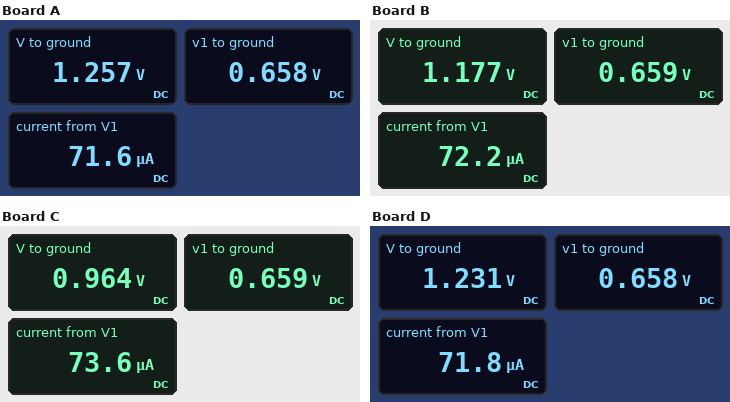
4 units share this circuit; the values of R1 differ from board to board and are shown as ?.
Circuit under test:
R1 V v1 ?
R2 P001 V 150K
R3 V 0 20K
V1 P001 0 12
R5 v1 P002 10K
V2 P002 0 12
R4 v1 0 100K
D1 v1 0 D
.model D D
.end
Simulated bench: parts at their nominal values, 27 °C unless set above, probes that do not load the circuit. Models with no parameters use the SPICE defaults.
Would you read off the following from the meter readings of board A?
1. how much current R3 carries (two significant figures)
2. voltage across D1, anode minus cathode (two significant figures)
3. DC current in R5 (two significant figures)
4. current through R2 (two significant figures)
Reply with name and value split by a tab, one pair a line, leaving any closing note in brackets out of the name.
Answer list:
how much current R3 carries	63 µA
voltage across D1, anode minus cathode	660 mV
DC current in R5	1.1 mA
current through R2	72 µA
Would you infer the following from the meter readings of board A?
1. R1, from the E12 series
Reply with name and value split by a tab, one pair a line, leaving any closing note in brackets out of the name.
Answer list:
R1, from the E12 series	68 kΩ
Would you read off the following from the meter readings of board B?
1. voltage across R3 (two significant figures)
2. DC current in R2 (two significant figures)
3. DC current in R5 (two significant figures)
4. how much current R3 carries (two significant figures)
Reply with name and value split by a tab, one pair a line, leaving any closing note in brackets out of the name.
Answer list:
voltage across R3	1.2 V
DC current in R2	72 µA
DC current in R5	1.1 mA
how much current R3 carries	59 µA
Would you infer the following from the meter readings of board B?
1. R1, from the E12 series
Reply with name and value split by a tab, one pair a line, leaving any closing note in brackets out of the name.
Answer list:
R1, from the E12 series	39 kΩ
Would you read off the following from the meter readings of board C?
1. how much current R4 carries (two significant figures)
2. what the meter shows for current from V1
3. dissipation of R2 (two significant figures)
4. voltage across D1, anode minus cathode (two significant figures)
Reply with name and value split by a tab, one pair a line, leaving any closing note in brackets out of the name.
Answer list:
how much current R4 carries	6.6 µA
what the meter shows for current from V1	73.6 µA
dissipation of R2	810 µW
voltage across D1, anode minus cathode	660 mV
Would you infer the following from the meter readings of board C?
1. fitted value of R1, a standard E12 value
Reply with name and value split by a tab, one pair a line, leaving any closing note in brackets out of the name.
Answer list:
fitted value of R1, a standard E12 value	12 kΩ
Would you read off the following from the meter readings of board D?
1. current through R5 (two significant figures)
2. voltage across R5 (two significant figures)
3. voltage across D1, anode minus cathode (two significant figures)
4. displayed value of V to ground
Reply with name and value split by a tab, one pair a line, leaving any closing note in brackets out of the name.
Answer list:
current through R5	1.1 mA
voltage across R5	11 V
voltage across D1, anode minus cathode	660 mV
displayed value of V to ground	1.231 V
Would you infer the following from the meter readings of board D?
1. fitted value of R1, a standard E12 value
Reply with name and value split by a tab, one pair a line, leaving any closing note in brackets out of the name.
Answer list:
fitted value of R1, a standard E12 value	56 kΩ
